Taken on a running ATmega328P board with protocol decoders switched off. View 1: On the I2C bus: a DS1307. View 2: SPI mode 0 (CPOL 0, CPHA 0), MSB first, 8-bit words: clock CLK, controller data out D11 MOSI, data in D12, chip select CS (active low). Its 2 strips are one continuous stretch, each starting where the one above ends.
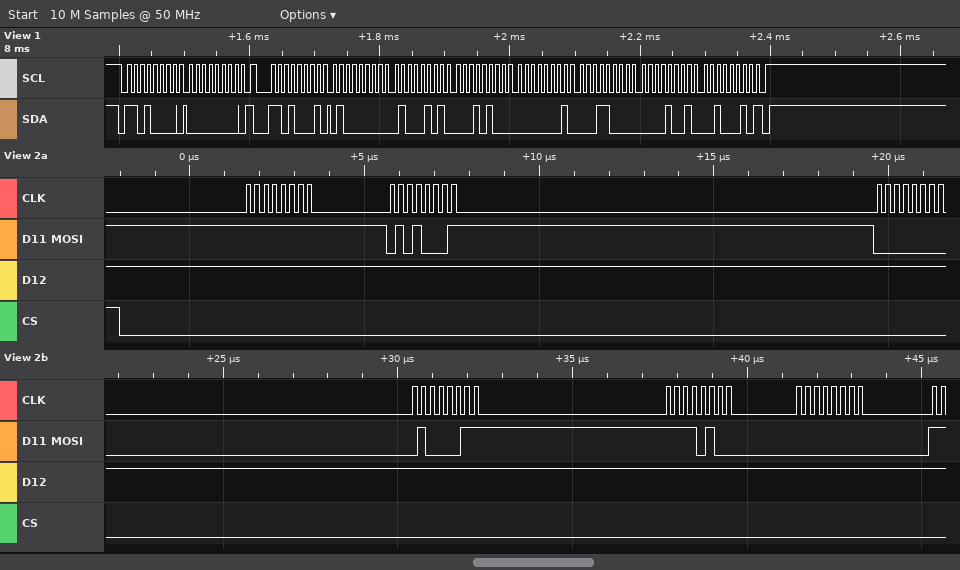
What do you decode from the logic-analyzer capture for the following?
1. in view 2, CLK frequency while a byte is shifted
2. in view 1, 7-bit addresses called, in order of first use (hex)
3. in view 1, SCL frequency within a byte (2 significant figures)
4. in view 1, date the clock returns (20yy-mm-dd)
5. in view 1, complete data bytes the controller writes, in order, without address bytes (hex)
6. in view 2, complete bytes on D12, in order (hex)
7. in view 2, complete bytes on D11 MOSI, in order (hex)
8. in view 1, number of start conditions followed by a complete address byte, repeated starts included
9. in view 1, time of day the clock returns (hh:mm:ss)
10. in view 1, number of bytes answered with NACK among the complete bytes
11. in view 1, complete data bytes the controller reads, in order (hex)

4 MHz
0x68
100 kHz
2022-09-18
00
FF FF FF FF FF FF
FF 51 00 43 F4 00
2
14:45:40
1
40 45 14 01 18 09 22
